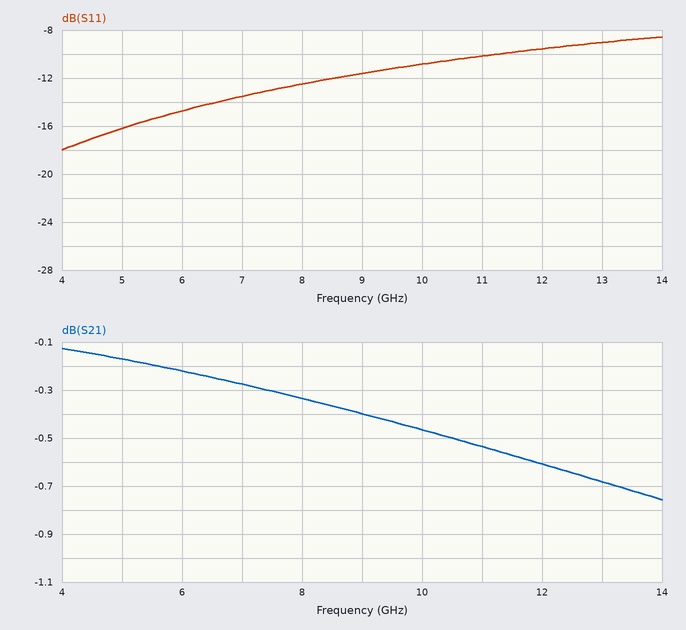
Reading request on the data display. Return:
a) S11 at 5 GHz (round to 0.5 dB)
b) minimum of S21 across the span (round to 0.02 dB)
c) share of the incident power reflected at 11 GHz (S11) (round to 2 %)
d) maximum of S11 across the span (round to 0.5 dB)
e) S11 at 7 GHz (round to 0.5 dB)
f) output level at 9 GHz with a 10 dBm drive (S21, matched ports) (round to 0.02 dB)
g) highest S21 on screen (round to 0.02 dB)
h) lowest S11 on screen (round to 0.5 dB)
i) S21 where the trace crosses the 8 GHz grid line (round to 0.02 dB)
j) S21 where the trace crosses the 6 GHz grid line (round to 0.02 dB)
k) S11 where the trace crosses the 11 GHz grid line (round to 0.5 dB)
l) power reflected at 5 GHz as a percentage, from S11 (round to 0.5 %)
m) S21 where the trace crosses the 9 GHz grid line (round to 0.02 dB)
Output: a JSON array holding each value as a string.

["-16.0 dB", "-0.76 dB", "10 %", "-8.5 dB", "-13.5 dB", "9.60 dBm", "-0.12 dB", "-18.0 dB", "-0.34 dB", "-0.22 dB", "-10.0 dB", "2.5 %", "-0.40 dB"]
